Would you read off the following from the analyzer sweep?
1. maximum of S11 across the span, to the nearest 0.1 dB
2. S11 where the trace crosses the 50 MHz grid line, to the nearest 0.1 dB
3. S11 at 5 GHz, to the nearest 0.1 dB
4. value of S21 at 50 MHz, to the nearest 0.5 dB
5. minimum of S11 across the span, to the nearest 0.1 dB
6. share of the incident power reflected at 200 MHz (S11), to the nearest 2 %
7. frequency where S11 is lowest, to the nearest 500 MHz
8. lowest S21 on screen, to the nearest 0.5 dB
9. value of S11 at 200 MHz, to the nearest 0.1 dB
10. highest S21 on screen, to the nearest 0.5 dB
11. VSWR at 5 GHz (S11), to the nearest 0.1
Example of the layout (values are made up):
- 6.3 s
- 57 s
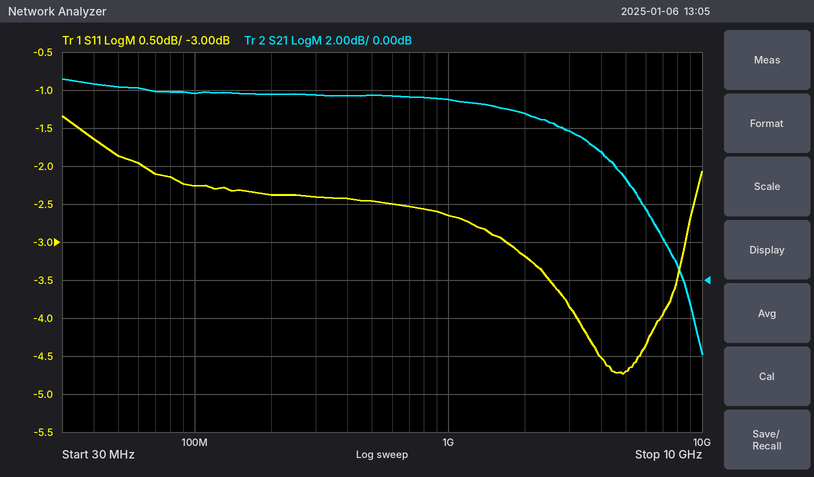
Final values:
- -1.3 dB
- -1.9 dB
- -4.7 dB
- 10.0 dB
- -4.7 dB
- 58 %
- 5.0 GHz
- -4.0 dB
- -2.4 dB
- 10.5 dB
- 3.8
